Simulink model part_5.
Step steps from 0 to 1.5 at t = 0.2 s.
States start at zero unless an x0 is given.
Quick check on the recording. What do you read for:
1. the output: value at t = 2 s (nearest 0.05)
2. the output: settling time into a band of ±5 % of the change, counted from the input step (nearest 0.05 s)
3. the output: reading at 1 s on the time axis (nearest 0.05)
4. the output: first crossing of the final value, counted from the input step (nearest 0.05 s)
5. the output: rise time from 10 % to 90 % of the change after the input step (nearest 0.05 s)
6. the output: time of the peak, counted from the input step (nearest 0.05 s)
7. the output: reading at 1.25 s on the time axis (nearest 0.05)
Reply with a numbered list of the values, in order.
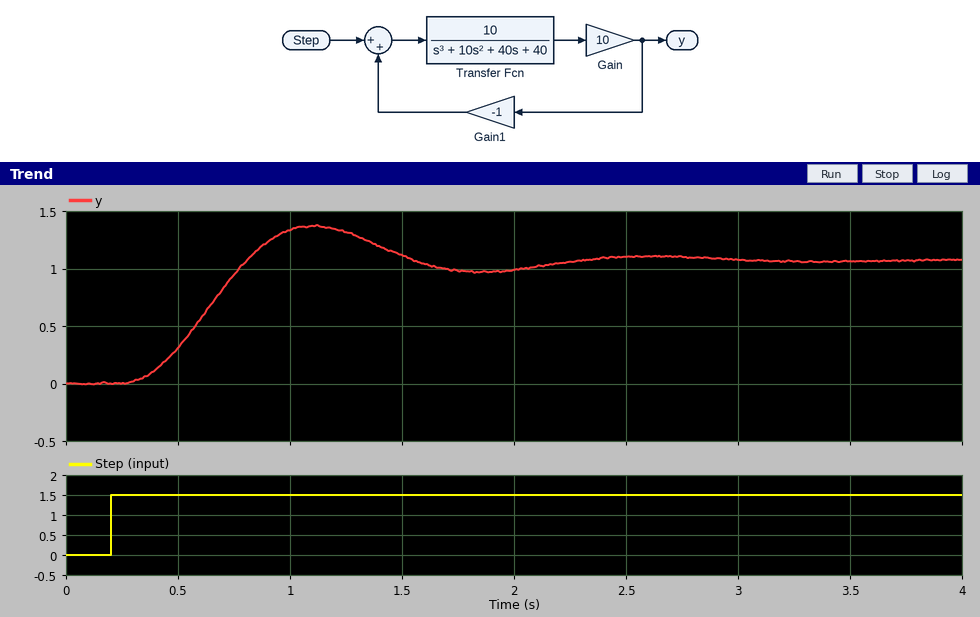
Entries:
1. 1.00
2. 1.90 s
3. 1.35
4. 0.60 s
5. 0.35 s
6. 0.90 s
7. 1.30
